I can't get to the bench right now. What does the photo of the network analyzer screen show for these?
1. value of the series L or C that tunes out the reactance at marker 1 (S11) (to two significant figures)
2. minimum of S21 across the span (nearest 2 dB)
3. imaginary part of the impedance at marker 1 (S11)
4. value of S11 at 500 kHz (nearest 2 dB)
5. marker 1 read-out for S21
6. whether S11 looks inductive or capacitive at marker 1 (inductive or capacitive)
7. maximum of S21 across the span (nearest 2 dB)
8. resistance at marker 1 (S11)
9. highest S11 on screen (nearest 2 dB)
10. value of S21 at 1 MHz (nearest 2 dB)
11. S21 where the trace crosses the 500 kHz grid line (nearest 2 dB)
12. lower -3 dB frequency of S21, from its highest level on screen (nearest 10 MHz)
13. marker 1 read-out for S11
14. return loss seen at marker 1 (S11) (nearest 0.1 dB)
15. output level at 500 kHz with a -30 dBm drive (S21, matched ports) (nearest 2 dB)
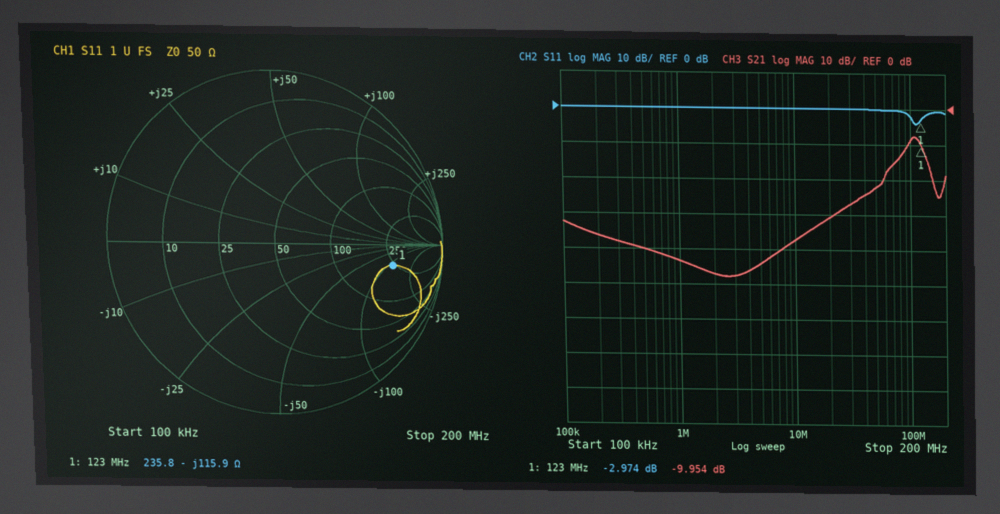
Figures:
150 nH
-48 dB
-115.9 Ω
0 dB
-9.954 dB
capacitive
-8 dB
235.8 Ω
0 dB
-44 dB
-40 dB
90 MHz
-2.974 dB
3.0 dB
-70 dBm
